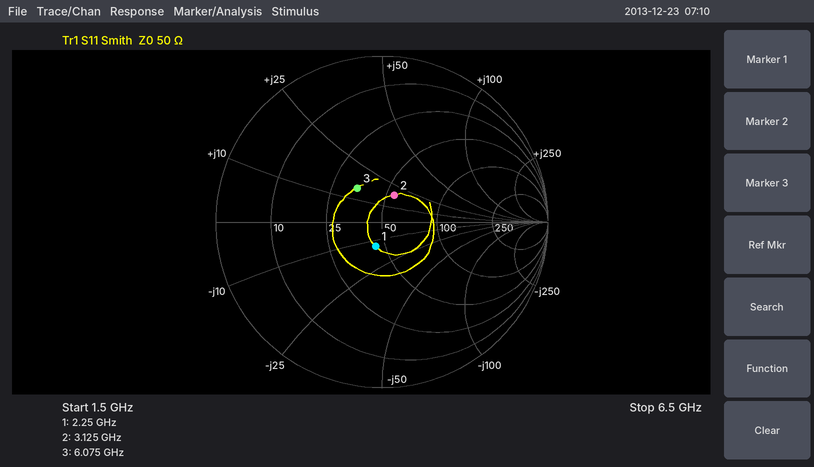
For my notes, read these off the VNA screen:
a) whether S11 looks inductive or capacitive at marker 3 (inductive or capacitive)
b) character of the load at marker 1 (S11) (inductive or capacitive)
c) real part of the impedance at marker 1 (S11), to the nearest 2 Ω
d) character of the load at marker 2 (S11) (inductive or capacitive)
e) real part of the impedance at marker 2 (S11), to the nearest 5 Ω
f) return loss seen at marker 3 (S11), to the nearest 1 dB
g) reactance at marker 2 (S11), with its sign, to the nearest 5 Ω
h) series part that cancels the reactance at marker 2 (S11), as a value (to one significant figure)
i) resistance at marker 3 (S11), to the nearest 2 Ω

inductive
capacitive
44 Ω
inductive
55 Ω
12 dB
+20 Ω
3 pF
34 Ω
